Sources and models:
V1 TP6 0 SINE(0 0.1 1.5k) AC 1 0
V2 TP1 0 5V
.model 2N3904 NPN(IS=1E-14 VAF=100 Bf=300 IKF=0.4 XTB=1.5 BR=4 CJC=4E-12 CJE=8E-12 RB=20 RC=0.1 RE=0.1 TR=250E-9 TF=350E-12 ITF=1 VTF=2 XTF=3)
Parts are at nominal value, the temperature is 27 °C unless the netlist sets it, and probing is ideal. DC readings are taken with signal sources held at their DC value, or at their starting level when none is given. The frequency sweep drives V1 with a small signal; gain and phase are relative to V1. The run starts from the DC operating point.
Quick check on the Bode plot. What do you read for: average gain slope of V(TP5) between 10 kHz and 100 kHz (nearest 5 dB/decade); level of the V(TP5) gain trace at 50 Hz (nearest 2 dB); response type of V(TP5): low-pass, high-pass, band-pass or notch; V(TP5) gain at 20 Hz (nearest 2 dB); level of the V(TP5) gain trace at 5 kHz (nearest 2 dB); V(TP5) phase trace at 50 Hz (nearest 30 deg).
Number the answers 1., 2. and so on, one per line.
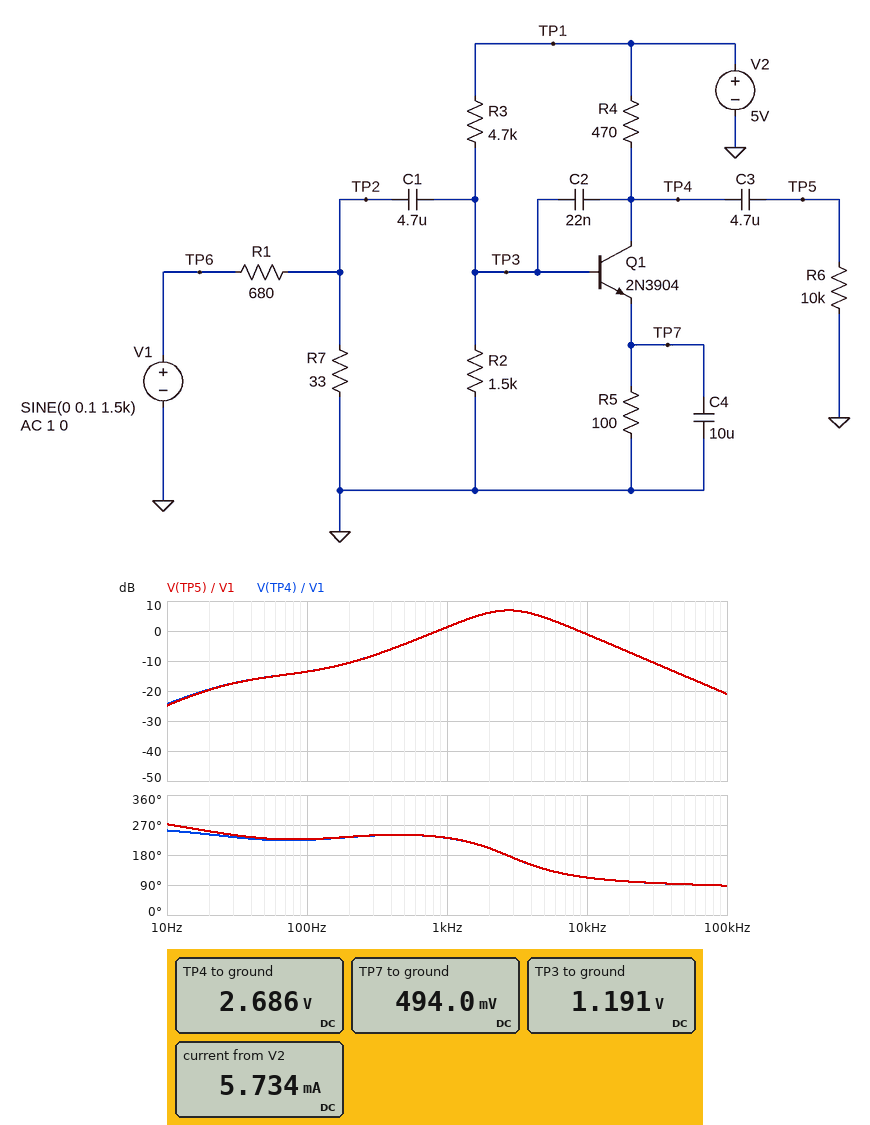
1. -20 dB/decade
2. -16 dB
3. band-pass
4. -20 dB
5. 4 dB
6. 240 deg
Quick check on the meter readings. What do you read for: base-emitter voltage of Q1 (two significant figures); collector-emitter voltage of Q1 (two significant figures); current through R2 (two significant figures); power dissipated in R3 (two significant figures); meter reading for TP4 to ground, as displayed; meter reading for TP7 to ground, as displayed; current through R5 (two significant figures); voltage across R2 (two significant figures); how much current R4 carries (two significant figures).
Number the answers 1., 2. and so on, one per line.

1. 700 mV
2. 2.2 V
3. 790 µA
4. 3.1 mW
5. 2.686 V
6. 494.0 mV
7. 4.9 mA
8. 1.2 V
9. 4.9 mA
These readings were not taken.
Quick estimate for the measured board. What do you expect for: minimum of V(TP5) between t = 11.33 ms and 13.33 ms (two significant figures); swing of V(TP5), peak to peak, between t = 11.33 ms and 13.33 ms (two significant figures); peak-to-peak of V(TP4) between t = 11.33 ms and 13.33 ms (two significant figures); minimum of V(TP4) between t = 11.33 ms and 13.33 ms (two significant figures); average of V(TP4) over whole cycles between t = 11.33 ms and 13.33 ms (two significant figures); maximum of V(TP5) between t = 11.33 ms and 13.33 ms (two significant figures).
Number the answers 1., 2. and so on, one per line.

1. -170 mV
2. 330 mV
3. 330 mV
4. 2.5 V
5. 2.7 V
6. 160 mV
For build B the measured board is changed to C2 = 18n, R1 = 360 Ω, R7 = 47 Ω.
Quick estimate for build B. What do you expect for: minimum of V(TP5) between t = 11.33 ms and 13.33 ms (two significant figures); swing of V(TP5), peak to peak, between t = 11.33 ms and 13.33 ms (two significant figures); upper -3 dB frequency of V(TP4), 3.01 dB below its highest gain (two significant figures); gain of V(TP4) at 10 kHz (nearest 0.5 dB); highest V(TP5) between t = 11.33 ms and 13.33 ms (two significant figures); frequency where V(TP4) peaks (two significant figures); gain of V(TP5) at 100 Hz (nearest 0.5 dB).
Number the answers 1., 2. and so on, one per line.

1. -440 mV
2. 850 mV
3. 5.1 kHz
4. 6.5 dB
5. 410 mV
6. 2.7 kHz
7. -5.5 dB
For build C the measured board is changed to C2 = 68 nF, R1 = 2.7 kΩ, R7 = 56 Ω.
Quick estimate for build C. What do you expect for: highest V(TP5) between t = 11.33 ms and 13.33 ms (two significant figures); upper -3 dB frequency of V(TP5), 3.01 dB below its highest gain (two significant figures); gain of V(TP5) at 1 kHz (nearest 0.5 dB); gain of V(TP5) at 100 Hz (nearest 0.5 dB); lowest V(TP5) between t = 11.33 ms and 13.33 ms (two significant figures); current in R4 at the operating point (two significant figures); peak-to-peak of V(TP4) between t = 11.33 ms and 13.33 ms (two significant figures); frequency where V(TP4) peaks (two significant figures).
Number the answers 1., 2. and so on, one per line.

1. 49 mV
2. 2.2 kHz
3. -6.5 dB
4. -21.0 dB
5. -49 mV
6. 4.9 mA
7. 98 mV
8. 1.3 kHz
